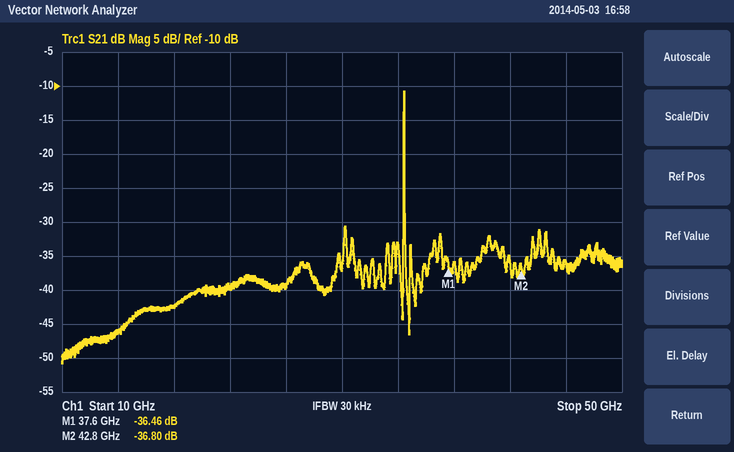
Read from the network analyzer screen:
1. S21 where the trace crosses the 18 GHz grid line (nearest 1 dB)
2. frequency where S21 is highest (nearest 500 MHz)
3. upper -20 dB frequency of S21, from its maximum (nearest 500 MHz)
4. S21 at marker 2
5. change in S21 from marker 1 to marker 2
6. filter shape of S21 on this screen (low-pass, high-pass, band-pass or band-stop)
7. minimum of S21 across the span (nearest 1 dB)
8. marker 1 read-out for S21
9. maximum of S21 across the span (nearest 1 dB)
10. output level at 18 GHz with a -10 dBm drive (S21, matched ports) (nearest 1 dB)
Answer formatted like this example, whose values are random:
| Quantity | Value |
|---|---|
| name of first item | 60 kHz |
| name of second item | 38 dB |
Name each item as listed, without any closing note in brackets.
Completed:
| Quantity | Value |
|---|---|
| S21 where the trace crosses the 18 GHz grid line | -42 dB |
| frequency where S21 is highest | 34.5 GHz |
| upper -20 dB frequency of S21, from its maximum | 34.5 GHz |
| S21 at marker 2 | -36.80 dB |
| change in S21 from marker 1 to marker 2 | -0.34 dB |
| filter shape of S21 on this screen | band-pass |
| minimum of S21 across the span | -51 dB |
| marker 1 read-out for S21 | -36.46 dB |
| maximum of S21 across the span | -11 dB |
| output level at 18 GHz with a -10 dBm drive (S21, matched ports) | -52 dBm |
